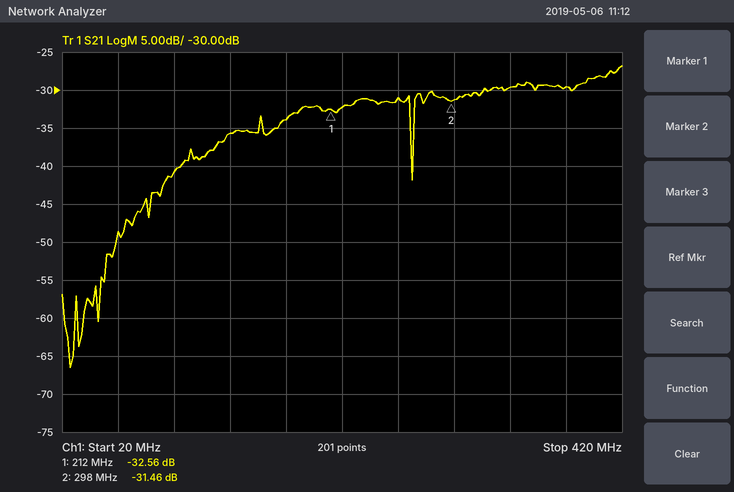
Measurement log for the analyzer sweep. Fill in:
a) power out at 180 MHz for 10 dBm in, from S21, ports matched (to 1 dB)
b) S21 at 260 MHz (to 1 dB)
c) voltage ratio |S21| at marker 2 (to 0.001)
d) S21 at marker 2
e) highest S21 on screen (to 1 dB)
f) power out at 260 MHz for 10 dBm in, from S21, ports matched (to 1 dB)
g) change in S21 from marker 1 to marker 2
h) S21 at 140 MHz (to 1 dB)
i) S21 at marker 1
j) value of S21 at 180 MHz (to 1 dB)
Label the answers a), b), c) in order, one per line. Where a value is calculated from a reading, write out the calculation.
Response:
a) 10 dBm + (-34 dB) = -24 dBm
b) -31 dB
c) 10^(-31.46/20) ≈ 0.027
d) -31.46 dB
e) -27 dB
f) 10 dBm + (-31 dB) = -21 dBm
g) -31.46 − (-32.56) = 1.10 dB
h) -36 dB
i) -32.56 dB
j) -34 dB
